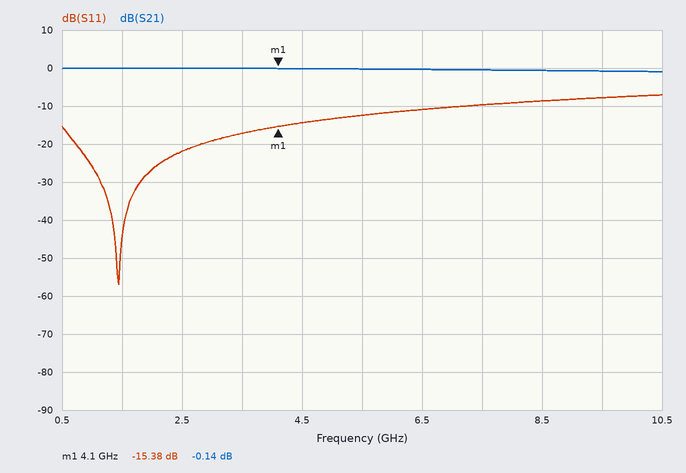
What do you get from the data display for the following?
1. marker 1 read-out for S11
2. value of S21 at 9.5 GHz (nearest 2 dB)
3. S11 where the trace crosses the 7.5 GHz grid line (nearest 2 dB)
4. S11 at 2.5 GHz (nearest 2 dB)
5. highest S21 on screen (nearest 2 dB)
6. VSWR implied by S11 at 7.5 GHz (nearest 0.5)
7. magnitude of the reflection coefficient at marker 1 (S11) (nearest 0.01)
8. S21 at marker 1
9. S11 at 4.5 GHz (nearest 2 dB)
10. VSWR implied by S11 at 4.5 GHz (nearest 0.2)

-15.38 dB
0 dB
-10 dB
-22 dB
0 dB
2.0
0.17
-0.14 dB
-14 dB
1.4
